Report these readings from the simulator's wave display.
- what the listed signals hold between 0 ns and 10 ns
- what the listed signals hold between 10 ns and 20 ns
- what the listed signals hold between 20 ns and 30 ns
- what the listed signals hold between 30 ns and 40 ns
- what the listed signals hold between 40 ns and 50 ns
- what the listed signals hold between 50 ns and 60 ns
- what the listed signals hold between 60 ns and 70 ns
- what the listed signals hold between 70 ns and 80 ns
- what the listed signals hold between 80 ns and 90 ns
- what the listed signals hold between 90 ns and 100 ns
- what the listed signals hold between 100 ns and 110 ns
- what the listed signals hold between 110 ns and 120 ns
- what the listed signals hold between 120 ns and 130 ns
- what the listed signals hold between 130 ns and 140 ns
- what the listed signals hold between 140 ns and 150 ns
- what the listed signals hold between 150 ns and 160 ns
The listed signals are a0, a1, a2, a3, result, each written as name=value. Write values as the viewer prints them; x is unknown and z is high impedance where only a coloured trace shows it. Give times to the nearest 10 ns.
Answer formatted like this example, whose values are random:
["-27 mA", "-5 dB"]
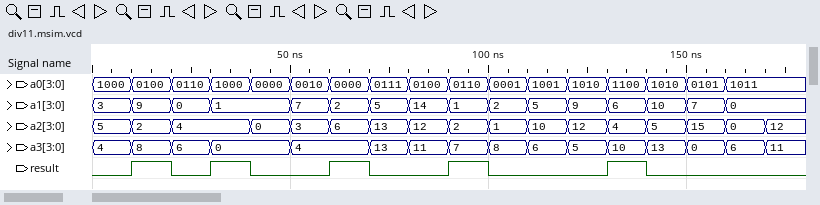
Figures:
["a0=1000, a1=3, a2=5, a3=4, result=0", "a0=0100, a1=9, a2=2, a3=8, result=1", "a0=0110, a1=0, a2=4, a3=6, result=0", "a0=1000, a1=1, a2=4, a3=0, result=1", "a0=0000, a1=1, a2=0, a3=0, result=0", "a0=0010, a1=7, a2=3, a3=4, result=0", "a0=0000, a1=2, a2=6, a3=4, result=1", "a0=0111, a1=5, a2=13, a3=13, result=0", "a0=0100, a1=14, a2=12, a3=11, result=0", "a0=0110, a1=1, a2=2, a3=7, result=1", "a0=0001, a1=2, a2=1, a3=8, result=0", "a0=1001, a1=5, a2=10, a3=6, result=0", "a0=1010, a1=9, a2=12, a3=5, result=0", "a0=1100, a1=6, a2=4, a3=10, result=1", "a0=1010, a1=10, a2=5, a3=13, result=0", "a0=0101, a1=7, a2=15, a3=0, result=0"]
